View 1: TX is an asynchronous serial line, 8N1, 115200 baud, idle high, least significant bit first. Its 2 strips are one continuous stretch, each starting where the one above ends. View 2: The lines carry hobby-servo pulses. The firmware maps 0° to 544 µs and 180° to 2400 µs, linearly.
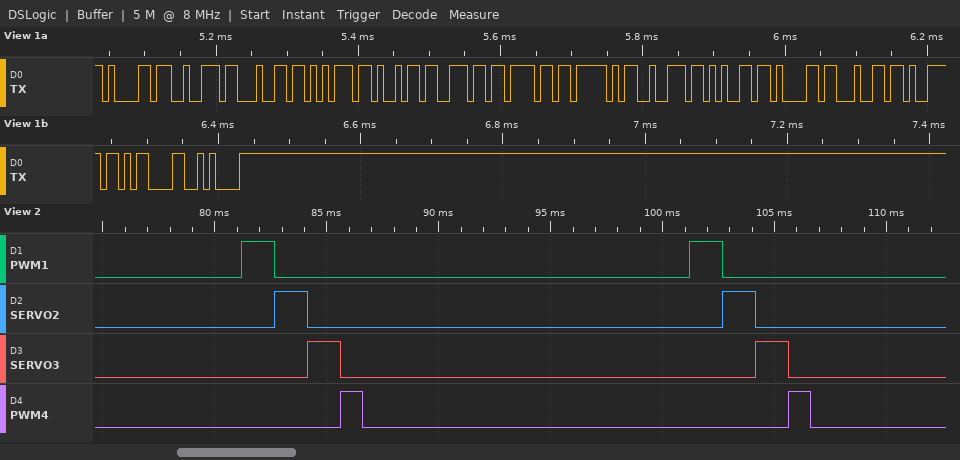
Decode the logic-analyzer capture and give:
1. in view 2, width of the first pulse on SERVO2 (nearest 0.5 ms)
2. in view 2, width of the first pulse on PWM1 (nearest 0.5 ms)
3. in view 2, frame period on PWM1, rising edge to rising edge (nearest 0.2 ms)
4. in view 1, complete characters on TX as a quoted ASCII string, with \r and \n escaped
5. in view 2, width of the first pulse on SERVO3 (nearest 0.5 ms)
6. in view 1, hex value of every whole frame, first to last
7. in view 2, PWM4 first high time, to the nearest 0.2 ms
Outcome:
1.5 ms
1.5 ms
20.0 ms
"arduino_ready\r\n"
1.5 ms
0x61 0x72 0x64 0x75 0x69 0x6E 0x6F 0x5F 0x72 0x65 0x61 0x64 0x79 0x0D 0x0A
1.0 ms
